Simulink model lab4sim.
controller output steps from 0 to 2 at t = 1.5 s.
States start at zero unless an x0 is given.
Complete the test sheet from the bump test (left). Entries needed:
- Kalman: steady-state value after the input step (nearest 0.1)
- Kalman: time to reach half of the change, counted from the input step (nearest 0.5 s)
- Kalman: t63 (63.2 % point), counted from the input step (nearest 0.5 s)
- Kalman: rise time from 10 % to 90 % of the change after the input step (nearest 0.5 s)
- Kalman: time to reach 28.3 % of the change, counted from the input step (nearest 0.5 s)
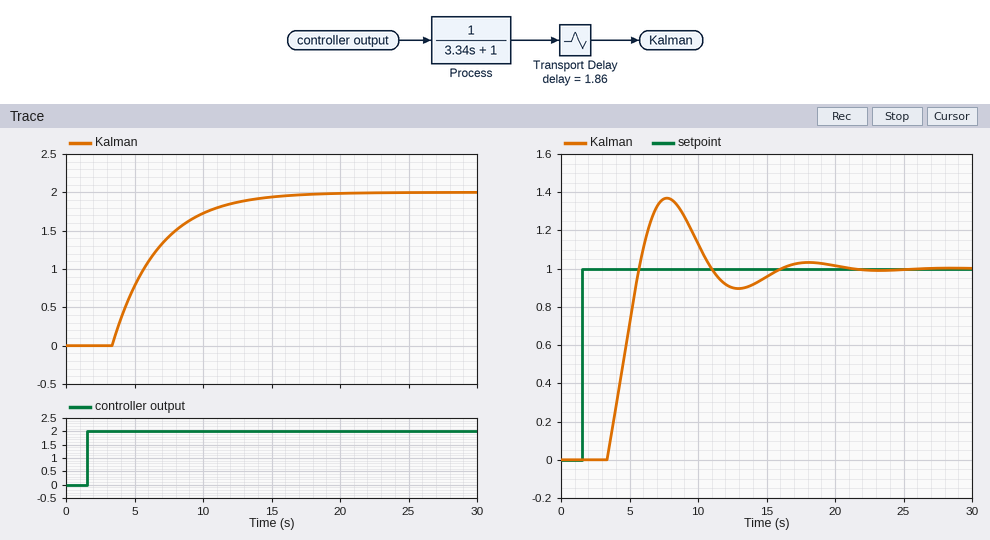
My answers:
2.0
4.0 s
5.0 s
7.5 s
3.0 s
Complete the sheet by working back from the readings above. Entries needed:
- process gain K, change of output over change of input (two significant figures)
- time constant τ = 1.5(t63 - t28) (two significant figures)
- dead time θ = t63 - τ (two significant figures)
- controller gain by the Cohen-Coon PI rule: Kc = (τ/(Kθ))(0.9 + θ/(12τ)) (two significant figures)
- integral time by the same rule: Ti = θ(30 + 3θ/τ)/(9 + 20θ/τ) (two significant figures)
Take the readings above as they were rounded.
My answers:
1.0
3.0 s
2.0 s
1.4
2.9 s
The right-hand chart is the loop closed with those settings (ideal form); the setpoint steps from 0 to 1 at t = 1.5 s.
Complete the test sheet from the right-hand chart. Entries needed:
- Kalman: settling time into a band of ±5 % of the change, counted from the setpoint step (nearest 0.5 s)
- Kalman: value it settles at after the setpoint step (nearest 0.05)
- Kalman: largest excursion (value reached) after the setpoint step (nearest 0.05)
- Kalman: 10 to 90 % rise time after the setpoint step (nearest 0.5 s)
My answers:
13.5 s
1.00
1.35
2.0 s
